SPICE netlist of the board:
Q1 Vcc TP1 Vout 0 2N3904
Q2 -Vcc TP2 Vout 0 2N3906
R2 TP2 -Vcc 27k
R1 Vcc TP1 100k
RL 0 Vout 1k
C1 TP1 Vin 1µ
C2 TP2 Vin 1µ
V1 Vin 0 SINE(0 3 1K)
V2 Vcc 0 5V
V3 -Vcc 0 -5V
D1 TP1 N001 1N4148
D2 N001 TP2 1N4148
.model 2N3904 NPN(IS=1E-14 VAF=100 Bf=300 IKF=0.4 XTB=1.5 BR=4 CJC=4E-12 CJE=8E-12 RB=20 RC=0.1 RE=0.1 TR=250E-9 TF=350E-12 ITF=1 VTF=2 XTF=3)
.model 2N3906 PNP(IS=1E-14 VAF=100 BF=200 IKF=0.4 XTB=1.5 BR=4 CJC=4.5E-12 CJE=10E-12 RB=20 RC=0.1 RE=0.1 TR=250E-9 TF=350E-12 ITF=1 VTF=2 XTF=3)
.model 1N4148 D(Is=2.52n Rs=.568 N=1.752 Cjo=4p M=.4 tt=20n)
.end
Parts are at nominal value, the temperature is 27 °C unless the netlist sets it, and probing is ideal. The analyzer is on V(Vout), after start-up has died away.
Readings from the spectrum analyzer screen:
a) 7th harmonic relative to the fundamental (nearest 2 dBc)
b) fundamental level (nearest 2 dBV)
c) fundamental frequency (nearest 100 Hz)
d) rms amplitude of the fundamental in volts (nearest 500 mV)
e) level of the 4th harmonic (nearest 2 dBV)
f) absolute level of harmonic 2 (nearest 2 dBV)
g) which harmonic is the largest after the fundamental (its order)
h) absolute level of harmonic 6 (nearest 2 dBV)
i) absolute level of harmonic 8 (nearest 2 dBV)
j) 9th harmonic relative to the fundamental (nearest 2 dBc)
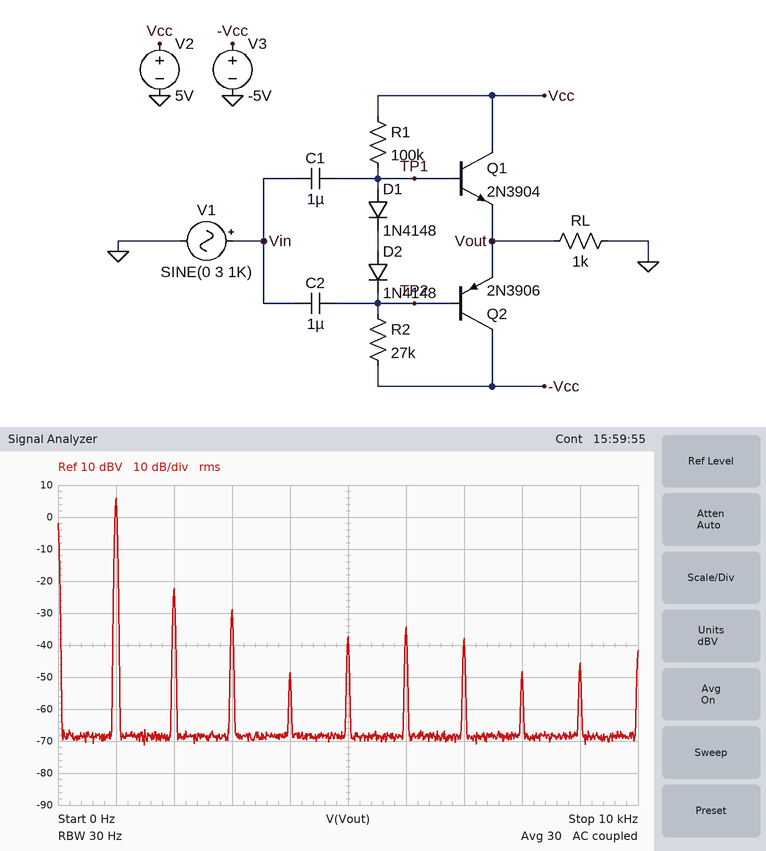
-44 dBc
6 dBV
1.0 kHz
2.0 V
-48 dBV
-22 dBV
2
-34 dBV
-48 dBV
-52 dBc
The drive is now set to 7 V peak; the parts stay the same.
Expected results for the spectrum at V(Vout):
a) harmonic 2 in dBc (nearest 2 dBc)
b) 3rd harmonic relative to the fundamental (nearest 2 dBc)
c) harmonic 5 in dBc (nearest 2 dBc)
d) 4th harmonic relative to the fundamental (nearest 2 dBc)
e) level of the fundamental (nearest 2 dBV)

-40 dBc
-16 dBc
-22 dBc
-44 dBc
10 dBV
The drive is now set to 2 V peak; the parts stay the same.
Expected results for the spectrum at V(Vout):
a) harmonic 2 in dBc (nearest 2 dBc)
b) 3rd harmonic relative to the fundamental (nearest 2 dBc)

-46 dBc
-54 dBc
